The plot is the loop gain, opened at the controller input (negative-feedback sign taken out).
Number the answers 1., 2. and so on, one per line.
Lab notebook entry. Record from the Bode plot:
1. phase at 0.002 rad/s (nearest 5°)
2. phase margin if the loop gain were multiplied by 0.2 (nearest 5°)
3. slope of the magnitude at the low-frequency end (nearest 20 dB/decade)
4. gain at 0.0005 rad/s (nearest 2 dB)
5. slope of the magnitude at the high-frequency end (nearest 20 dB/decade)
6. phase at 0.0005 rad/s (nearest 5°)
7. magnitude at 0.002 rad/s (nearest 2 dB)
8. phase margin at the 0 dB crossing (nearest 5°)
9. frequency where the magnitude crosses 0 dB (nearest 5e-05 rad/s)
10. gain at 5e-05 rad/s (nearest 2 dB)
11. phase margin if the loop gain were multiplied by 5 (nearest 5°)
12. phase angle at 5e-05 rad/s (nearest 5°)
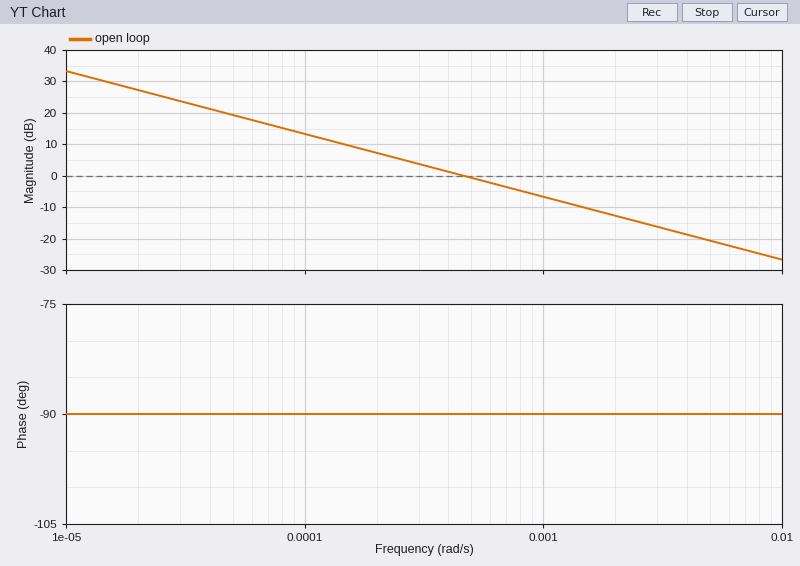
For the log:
1. -90°
2. 90°
3. -20 dB/decade
4. 0 dB
5. -20 dB/decade
6. -90°
7. -12 dB
8. 90°
9. 0.00045 rad/s
10. 20 dB
11. 90°
12. -90°
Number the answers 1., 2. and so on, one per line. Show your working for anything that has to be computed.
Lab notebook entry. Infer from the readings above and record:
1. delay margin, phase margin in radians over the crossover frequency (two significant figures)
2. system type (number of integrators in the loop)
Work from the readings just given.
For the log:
1. 90 × π / 180 / 0.00045 = 3500 s
2. 1
